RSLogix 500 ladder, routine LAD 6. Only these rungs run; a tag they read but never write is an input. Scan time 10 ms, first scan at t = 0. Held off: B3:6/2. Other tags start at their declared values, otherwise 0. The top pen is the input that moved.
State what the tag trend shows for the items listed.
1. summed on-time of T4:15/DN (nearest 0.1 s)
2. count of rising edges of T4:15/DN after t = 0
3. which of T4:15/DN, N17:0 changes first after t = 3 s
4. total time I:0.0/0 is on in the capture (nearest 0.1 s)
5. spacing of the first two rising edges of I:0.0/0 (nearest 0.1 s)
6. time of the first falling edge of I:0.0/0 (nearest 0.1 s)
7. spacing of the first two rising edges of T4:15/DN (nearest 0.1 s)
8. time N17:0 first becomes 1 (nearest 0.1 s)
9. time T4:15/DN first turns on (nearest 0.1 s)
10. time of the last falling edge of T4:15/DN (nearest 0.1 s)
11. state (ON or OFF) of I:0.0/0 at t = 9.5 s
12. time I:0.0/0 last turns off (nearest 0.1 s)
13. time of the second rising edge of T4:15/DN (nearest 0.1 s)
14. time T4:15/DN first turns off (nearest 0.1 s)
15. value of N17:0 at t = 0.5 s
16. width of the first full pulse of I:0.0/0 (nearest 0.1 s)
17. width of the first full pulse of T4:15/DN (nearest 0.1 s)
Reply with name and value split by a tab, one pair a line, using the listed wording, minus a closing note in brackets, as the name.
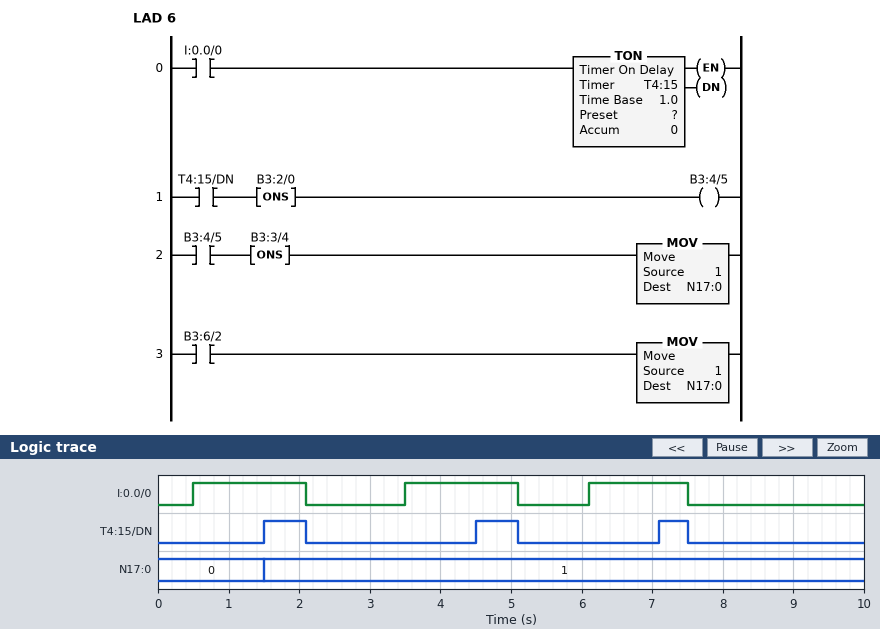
summed on-time of T4:15/DN	1.6 s
count of rising edges of T4:15/DN after t = 0	3
which of T4:15/DN, N17:0 changes first after t = 3 s	T4:15/DN
total time I:0.0/0 is on in the capture	4.6 s
spacing of the first two rising edges of I:0.0/0	3.0 s
time of the first falling edge of I:0.0/0	2.1 s
spacing of the first two rising edges of T4:15/DN	3.0 s
time N17:0 first becomes 1	1.5 s
time T4:15/DN first turns on	1.5 s
time of the last falling edge of T4:15/DN	7.5 s
state (ON or OFF) of I:0.0/0 at t = 9.5 s	OFF
time I:0.0/0 last turns off	7.5 s
time of the second rising edge of T4:15/DN	4.5 s
time T4:15/DN first turns off	2.1 s
value of N17:0 at t = 0.5 s	0
width of the first full pulse of I:0.0/0	1.6 s
width of the first full pulse of T4:15/DN	0.6 s
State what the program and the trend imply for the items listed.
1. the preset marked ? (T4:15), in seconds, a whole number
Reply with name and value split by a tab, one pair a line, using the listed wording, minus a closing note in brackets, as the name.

the preset marked ? (T4:15), in seconds, a whole number	1 s
